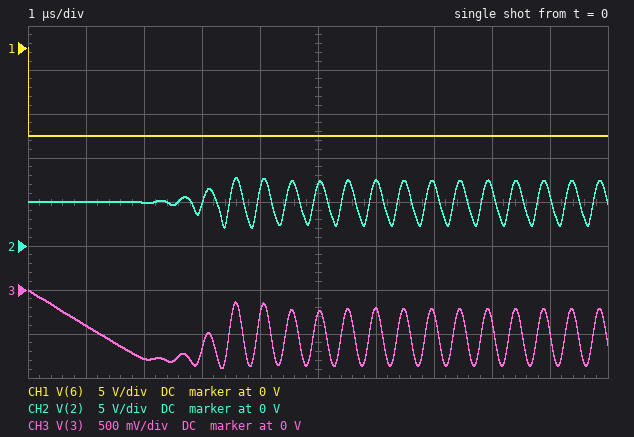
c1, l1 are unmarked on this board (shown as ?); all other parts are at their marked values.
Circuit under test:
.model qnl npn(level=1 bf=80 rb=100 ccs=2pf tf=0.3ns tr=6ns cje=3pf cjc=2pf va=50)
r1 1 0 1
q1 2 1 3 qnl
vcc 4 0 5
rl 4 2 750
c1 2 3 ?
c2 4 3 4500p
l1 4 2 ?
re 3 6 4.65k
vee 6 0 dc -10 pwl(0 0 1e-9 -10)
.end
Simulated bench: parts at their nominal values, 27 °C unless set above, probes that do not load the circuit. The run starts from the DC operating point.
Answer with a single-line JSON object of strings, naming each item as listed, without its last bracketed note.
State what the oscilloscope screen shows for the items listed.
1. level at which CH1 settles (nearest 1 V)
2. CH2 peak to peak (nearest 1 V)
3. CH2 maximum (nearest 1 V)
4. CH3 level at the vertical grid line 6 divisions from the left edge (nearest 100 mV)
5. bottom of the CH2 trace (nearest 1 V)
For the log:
{"level at which CH1 settles": "-10 V", "CH2 peak to peak": "6 V", "CH2 maximum": "8 V", "CH3 level at the vertical grid line 6 divisions from the left edge": "-200 mV", "bottom of the CH2 trace": "2 V"}
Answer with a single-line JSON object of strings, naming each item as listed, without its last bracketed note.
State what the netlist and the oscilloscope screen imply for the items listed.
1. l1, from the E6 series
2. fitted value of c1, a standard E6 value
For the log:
{"l1, from the E6 series": "10 µH", "fitted value of c1, a standard E6 value": "680 pF"}
